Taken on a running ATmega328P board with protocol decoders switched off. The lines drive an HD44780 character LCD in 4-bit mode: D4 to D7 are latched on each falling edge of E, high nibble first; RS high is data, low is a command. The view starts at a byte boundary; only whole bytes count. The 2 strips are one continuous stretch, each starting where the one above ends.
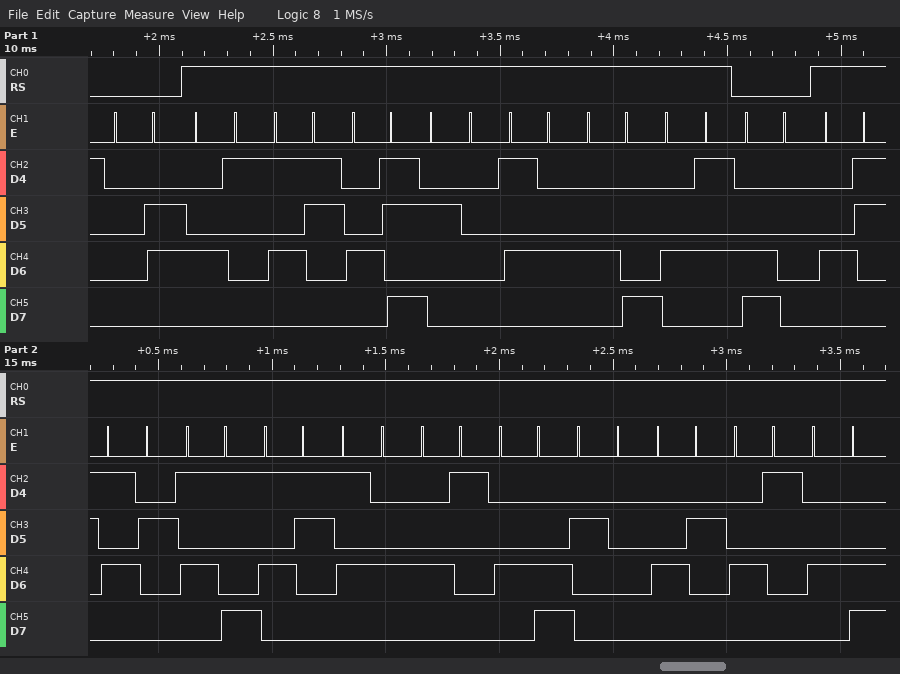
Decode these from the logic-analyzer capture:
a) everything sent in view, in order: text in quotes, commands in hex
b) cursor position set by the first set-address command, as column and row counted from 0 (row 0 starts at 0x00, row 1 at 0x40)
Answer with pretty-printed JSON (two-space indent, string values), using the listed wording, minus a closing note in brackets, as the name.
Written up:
{
  "everything sent in view, in order: text in quotes, commands in hex": "0x06 \"ASK THE\" 0xC0 \"CRYSTAL BAL\"",
  "cursor position set by the first set-address command, as column and row counted from 0": "column 0, row 1"
}
